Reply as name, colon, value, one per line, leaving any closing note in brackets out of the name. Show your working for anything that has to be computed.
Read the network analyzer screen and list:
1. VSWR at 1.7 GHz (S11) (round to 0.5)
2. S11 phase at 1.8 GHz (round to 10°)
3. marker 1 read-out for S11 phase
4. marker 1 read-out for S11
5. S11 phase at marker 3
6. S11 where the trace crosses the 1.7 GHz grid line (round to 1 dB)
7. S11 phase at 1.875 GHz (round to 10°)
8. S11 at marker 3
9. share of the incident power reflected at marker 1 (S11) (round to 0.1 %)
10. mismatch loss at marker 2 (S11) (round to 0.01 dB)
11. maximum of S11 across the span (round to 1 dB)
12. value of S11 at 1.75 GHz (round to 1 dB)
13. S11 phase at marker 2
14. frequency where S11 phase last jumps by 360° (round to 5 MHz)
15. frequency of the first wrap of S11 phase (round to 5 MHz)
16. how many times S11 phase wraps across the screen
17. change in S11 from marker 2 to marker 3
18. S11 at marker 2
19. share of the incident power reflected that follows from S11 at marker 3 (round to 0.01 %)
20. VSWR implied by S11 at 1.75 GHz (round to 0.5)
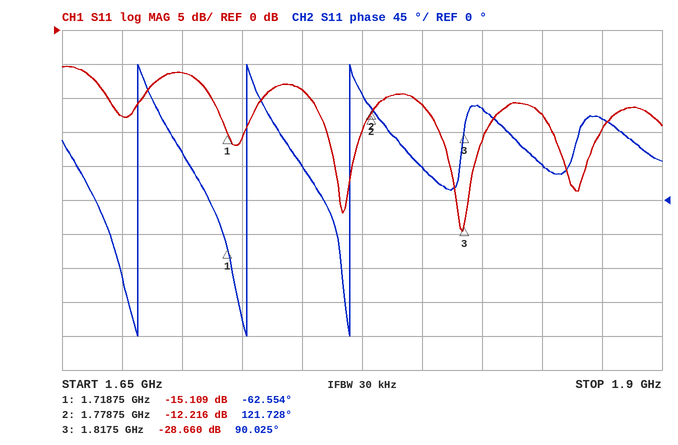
VSWR at 1.7 GHz (S11): |Γ| = 10^(-6/20) = 0.5012; VSWR = (1 + 0.5012)/(1 − 0.5012) ≈ 3.0
S11 phase at 1.8 GHz: 40°
marker 1 read-out for S11 phase: -62.554°
marker 1 read-out for S11: -15.109 dB
S11 phase at marker 3: 90.025°
S11 where the trace crosses the 1.7 GHz grid line: -6 dB
S11 phase at 1.875 GHz: 110°
S11 at marker 3: -28.660 dB
share of the incident power reflected at marker 1 (S11): 10^(-15.109/10) ≈ 3.1 %
mismatch loss at marker 2 (S11): −10 log10(1 − 10^(-12.216/10)) ≈ 0.27 dB
maximum of S11 across the span: -5 dB
value of S11 at 1.75 GHz: -9 dB
S11 phase at marker 2: 121.728°
frequency where S11 phase last jumps by 360°: 1.770 GHz
frequency of the first wrap of S11 phase: 1.680 GHz
how many times S11 phase wraps across the screen: 3
change in S11 from marker 2 to marker 3: -28.66 − (-12.216) = -16.444 dB
S11 at marker 2: -12.216 dB
share of the incident power reflected that follows from S11 at marker 3: 10^(-28.66/10) ≈ 0.14 %
VSWR implied by S11 at 1.75 GHz: |Γ| = 10^(-9/20) = 0.3548; VSWR = (1 + 0.3548)/(1 − 0.3548) ≈ 2.10, so 2.0 to the nearest 0.5
